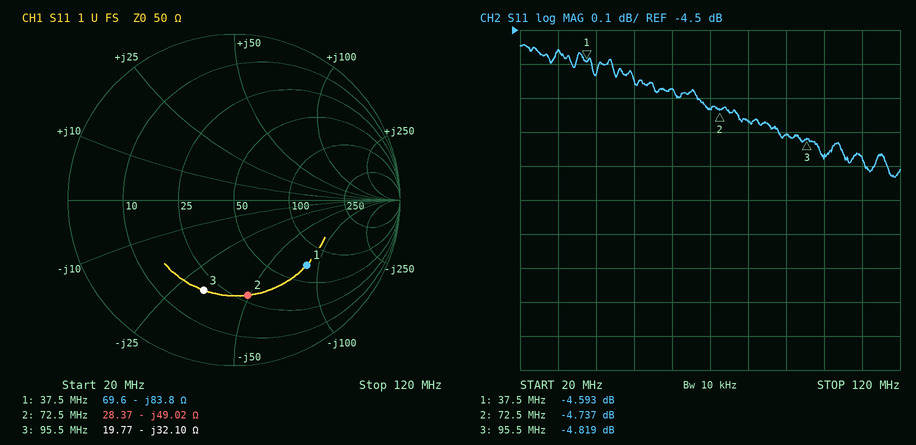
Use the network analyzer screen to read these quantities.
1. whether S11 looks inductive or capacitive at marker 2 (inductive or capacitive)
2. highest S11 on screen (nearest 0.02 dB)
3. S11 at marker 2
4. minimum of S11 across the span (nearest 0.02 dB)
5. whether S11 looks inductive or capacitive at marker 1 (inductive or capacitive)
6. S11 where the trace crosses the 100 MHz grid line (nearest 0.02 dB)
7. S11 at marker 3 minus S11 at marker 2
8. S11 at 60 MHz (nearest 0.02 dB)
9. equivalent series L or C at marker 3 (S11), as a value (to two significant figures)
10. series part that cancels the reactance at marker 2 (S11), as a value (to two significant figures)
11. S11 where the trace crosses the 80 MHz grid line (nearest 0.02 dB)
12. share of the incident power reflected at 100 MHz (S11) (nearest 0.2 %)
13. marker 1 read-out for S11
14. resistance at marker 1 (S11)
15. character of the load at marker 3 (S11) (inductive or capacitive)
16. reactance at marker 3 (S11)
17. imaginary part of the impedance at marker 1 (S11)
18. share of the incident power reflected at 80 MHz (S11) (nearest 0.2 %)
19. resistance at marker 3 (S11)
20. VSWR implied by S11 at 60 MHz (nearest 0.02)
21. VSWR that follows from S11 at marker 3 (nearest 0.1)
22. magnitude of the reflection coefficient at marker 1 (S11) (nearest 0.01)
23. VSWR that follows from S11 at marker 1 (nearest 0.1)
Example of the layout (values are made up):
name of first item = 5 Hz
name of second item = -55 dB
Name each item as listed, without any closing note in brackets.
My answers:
whether S11 looks inductive or capacitive at marker 2 = capacitive
highest S11 on screen = -4.54 dB
S11 at marker 2 = -4.737 dB
minimum of S11 across the span = -4.94 dB
whether S11 looks inductive or capacitive at marker 1 = capacitive
S11 where the trace crosses the 100 MHz grid line = -4.88 dB
S11 at marker 3 minus S11 at marker 2 = -0.082 dB
S11 at 60 MHz = -4.68 dB
equivalent series L or C at marker 3 (S11), as a value = 52 pF
series part that cancels the reactance at marker 2 (S11), as a value = 110 nH
S11 where the trace crosses the 80 MHz grid line = -4.76 dB
share of the incident power reflected at 100 MHz (S11) = 32.6 %
marker 1 read-out for S11 = -4.593 dB
resistance at marker 1 = 69.6 Ω
character of the load at marker 3 (S11) = capacitive
reactance at marker 3 = -32.10 Ω
imaginary part of the impedance at marker 1 = -83.8 Ω
share of the incident power reflected at 80 MHz (S11) = 33.4 %
resistance at marker 3 = 19.77 Ω
VSWR implied by S11 at 60 MHz = 3.80
VSWR that follows from S11 at marker 3 = 3.7
magnitude of the reflection coefficient at marker 1 (S11) = 0.59
VSWR that follows from S11 at marker 1 = 3.9
